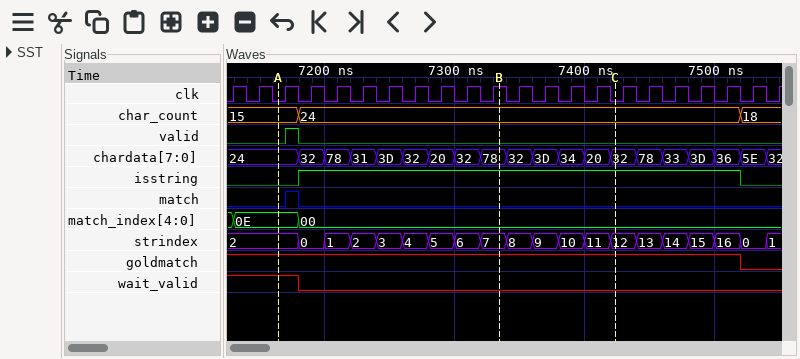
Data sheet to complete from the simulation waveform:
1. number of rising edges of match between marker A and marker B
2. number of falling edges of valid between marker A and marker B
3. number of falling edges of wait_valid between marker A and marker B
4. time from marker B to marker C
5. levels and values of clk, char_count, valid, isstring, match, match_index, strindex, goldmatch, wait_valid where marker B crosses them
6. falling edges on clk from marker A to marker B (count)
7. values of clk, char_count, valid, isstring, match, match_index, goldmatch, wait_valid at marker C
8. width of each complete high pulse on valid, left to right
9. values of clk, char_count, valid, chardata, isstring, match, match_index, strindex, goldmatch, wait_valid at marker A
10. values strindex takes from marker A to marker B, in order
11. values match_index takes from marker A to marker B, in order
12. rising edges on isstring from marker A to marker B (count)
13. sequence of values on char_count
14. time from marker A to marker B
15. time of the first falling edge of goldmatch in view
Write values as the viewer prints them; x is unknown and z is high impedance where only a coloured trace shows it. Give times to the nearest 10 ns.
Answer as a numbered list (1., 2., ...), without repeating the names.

1. 1
2. 1
3. 1
4. 90 ns
5. clk=1, char_count=24, valid=0, isstring=1, match=0, match_index=00, strindex=7, goldmatch=1, wait_valid=0
6. 8
7. clk=0, char_count=24, valid=0, isstring=1, match=0, match_index=00, goldmatch=1, wait_valid=0
8. 10 ns
9. clk=0, char_count=15, valid=0, chardata=24, isstring=0, match=0, match_index=0E, strindex=2, goldmatch=1, wait_valid=1
10. 2, 0, 1, 2, 3, 4, 5, 6, 7
11. 0E, 00
12. 1
13. 15, 24, 18
14. 170 ns
15. 7520 ns
